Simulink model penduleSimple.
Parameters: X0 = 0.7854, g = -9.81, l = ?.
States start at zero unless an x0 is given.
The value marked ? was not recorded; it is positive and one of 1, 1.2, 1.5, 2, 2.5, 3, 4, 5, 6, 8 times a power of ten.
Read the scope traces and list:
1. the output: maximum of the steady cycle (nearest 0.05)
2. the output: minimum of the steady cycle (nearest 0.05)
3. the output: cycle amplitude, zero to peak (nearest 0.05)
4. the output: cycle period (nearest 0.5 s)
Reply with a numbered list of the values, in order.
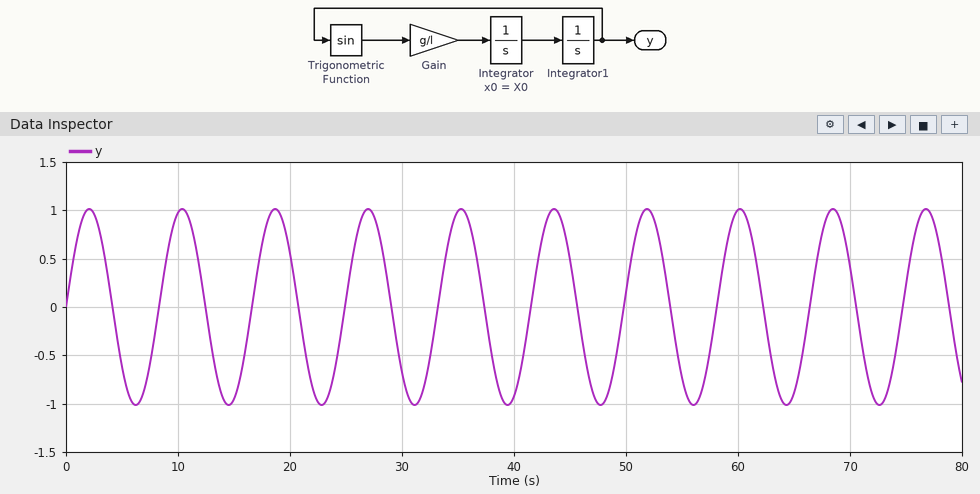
1. 1.00
2. -1.00
3. 1.00
4. 8.5 s
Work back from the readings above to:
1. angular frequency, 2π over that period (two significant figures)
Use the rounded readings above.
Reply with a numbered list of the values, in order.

1. 0.74 rad/s
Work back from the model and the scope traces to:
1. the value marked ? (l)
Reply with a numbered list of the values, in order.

1. 15
